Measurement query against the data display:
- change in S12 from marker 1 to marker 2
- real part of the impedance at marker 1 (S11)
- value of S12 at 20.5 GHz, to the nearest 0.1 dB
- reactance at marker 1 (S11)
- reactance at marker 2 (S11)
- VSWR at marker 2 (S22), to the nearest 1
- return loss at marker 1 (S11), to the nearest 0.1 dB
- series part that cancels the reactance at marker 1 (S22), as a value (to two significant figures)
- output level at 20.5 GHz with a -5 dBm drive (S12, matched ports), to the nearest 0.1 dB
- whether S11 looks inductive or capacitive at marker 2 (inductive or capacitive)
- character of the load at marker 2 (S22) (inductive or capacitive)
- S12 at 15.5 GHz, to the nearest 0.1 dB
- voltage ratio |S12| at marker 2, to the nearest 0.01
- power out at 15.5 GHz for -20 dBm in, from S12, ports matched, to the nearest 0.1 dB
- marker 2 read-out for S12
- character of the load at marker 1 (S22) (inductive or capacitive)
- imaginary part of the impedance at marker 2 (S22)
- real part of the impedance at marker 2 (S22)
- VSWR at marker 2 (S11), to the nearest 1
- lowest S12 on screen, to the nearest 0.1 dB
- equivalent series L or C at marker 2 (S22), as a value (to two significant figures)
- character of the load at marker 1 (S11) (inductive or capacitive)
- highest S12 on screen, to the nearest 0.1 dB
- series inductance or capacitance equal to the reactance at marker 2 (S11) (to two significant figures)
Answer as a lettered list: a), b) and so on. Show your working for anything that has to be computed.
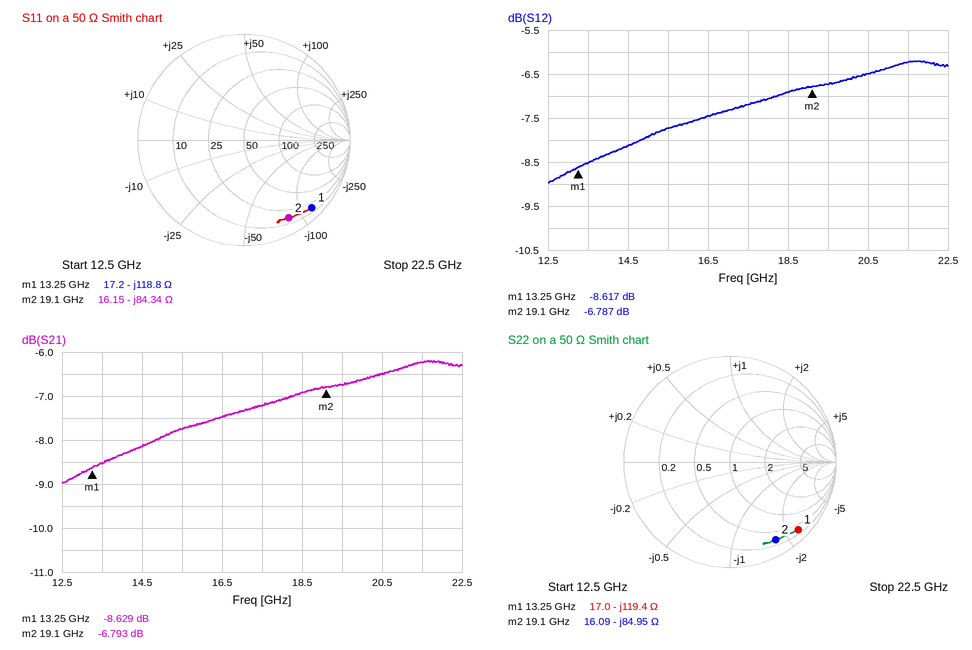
a) -6.787 − (-8.617) = 1.830 dB
b) 17.2 Ω
c) -6.5 dB
d) -118.8 Ω
e) -84.34 Ω
f) 12
g) 0.9 dB
h) L = 119.4 Ω/(2π × 13.25 GHz) ≈ 1.4 nH
i) -5 dBm + (-6.5 dB) = -11.5 dBm
j) capacitive
k) capacitive
l) -7.7 dB
m) 10^(-6.787/20) ≈ 0.46
n) -20 dBm + (-7.7 dB) = -27.7 dBm
o) -6.787 dB
p) capacitive
q) -84.95 Ω
r) 16.09 Ω
s) 12
t) -9.0 dB
u) C = 1/(2π × 19.1 GHz × 84.95 Ω) ≈ 98 fF
v) capacitive
w) -6.2 dB
x) C = 1/(2π × 19.1 GHz × 84.34 Ω) ≈ 99 fF
